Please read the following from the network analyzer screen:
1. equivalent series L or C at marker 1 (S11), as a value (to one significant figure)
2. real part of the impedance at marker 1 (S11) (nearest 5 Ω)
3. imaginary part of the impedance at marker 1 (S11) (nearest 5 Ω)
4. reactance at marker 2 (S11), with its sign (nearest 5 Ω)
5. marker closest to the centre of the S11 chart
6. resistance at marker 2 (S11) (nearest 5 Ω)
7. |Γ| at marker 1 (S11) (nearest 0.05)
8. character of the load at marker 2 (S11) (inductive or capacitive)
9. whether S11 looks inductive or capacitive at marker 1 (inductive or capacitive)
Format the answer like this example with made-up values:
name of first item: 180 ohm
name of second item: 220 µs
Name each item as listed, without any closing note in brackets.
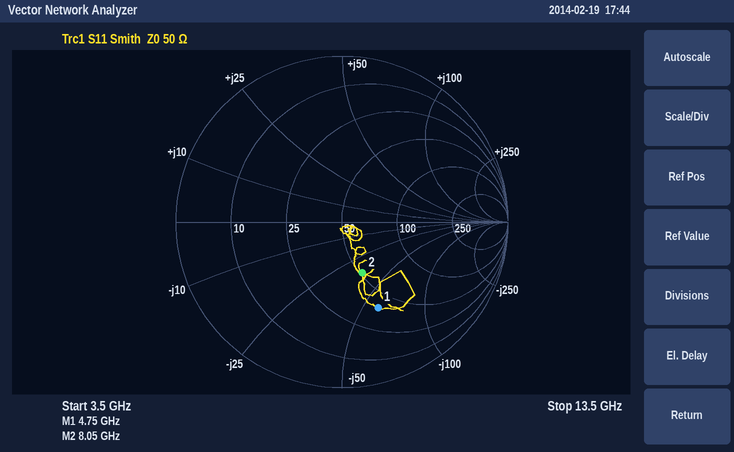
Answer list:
equivalent series L or C at marker 1 (S11), as a value: 600 fF
real part of the impedance at marker 1 (S11): 40 Ω
imaginary part of the impedance at marker 1 (S11): -60 Ω
reactance at marker 2 (S11), with its sign: -35 Ω
marker closest to the centre of the S11 chart: marker 2
resistance at marker 2 (S11): 50 Ω
|Γ| at marker 1 (S11): 0.55
character of the load at marker 2 (S11): capacitive
whether S11 looks inductive or capacitive at marker 1: capacitive
